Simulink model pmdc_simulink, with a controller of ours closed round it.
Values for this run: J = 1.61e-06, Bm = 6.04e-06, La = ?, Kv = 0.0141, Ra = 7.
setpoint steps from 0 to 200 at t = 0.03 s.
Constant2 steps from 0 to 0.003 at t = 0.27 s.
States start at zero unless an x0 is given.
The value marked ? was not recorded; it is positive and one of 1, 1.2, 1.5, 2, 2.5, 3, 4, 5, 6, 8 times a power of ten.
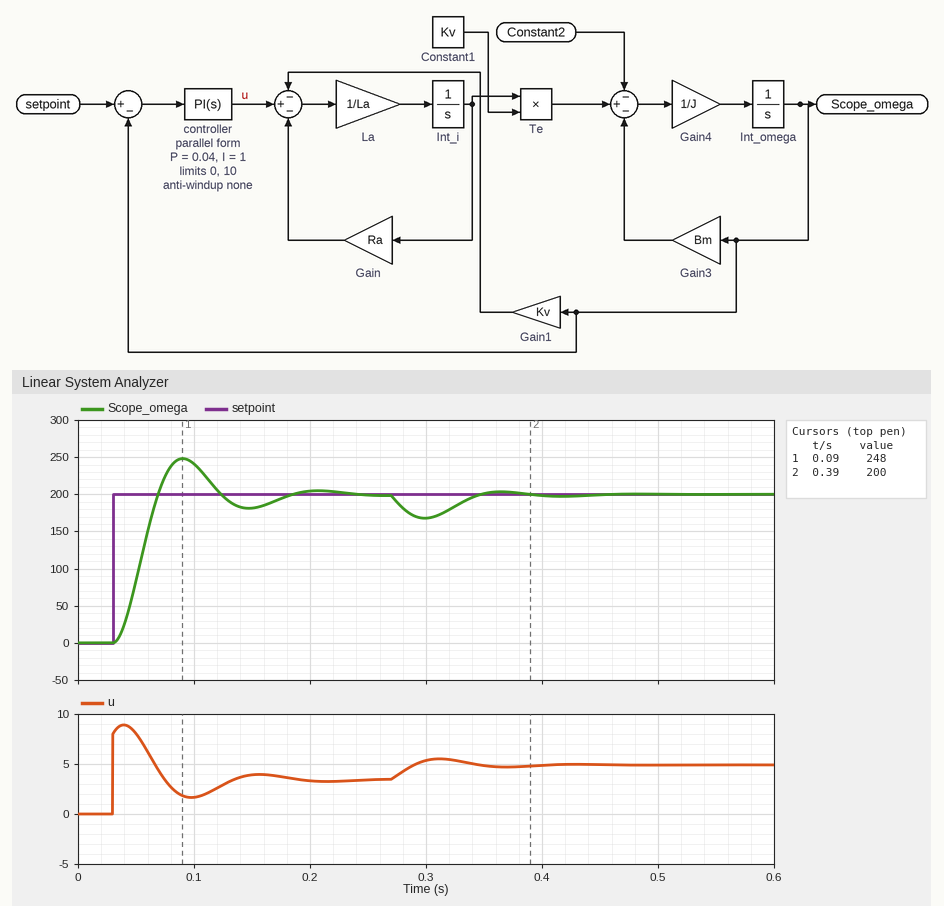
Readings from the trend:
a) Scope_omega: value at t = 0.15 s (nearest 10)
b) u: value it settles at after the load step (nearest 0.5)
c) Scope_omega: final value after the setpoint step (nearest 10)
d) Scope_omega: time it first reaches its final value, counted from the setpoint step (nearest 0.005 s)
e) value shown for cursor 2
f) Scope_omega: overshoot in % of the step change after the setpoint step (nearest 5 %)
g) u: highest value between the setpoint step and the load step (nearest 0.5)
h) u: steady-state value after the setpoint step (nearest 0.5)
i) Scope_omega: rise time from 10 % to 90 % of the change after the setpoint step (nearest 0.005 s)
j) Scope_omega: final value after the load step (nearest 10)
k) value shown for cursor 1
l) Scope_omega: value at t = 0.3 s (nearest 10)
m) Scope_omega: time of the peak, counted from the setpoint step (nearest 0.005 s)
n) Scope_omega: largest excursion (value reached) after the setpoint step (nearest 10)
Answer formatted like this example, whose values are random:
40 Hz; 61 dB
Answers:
180; 5.0; 200; 0.040 s; 200; 25 %; 9.0; 3.5; 0.025 s; 200; 248; 170; 0.060 s; 250
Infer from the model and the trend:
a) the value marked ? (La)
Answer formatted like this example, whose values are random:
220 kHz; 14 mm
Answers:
0.12
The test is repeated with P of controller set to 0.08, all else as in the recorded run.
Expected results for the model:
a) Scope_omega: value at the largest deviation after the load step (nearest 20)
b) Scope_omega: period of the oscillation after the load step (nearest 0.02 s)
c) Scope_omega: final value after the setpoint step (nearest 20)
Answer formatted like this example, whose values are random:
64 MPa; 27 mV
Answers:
180; 0.08 s; 200
